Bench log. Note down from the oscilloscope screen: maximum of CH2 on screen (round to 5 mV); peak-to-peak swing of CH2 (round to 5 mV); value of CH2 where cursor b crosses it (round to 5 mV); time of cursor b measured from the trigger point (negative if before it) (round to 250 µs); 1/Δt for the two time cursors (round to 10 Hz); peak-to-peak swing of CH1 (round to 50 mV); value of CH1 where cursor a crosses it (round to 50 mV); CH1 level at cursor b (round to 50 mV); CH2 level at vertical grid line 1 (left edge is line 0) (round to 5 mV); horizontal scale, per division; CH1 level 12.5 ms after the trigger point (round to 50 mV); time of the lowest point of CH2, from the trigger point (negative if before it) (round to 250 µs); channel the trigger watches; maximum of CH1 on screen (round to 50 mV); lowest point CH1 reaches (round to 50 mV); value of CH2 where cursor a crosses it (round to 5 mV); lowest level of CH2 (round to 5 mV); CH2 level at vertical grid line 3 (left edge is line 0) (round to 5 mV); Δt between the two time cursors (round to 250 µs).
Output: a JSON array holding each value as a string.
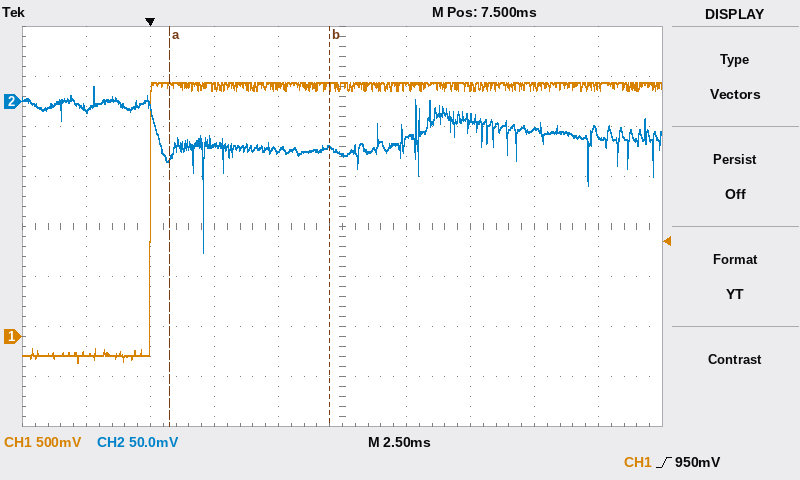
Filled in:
["15 mV", "165 mV", "-45 mV", "+7.00 ms", "160 Hz", "2.80 V", "2.50 V", "2.50 V", "-5 mV", "2.5 ms", "2.50 V", "+2.00 ms", "CH1", "2.55 V", "-250 mV", "-55 mV", "-150 mV", "-45 mV", "6.25 ms"]
